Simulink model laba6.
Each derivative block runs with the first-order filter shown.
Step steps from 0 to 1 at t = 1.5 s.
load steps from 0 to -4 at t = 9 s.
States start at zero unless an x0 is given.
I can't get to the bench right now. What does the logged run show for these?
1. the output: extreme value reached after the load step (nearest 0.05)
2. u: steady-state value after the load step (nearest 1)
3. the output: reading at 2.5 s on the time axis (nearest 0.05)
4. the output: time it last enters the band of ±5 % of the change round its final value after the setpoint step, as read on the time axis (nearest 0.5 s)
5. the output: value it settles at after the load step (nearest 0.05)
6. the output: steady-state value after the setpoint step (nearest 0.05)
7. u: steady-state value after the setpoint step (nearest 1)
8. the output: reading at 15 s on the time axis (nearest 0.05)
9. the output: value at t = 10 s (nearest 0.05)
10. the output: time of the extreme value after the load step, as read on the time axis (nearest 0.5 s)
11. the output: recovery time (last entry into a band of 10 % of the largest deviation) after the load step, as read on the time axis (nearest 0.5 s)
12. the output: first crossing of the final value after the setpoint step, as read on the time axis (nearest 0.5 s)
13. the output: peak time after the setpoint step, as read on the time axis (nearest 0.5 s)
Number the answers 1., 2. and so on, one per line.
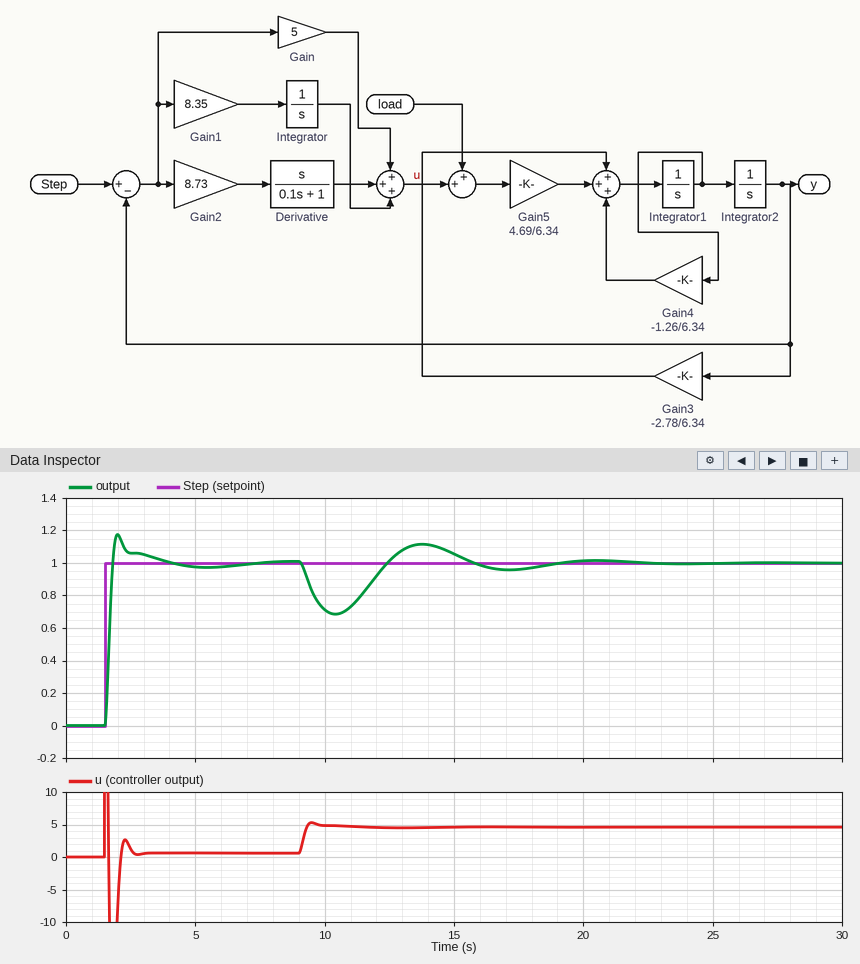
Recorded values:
1. 0.70
2. 5
3. 1.05
4. 3.0 s
5. 1.00
6. 1.00
7. 1
8. 1.05
9. 0.70
10. 10.5 s
11. 18.0 s
12. 2.0 s
13. 2.0 s
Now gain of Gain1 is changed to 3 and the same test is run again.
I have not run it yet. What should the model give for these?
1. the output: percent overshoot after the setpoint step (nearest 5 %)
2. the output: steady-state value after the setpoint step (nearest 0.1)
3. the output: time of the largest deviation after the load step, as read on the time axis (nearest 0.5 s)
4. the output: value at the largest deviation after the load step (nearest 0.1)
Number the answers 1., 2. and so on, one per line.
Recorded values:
1. 15 %
2. 1.0
3. 11.0 s
4. 0.6
